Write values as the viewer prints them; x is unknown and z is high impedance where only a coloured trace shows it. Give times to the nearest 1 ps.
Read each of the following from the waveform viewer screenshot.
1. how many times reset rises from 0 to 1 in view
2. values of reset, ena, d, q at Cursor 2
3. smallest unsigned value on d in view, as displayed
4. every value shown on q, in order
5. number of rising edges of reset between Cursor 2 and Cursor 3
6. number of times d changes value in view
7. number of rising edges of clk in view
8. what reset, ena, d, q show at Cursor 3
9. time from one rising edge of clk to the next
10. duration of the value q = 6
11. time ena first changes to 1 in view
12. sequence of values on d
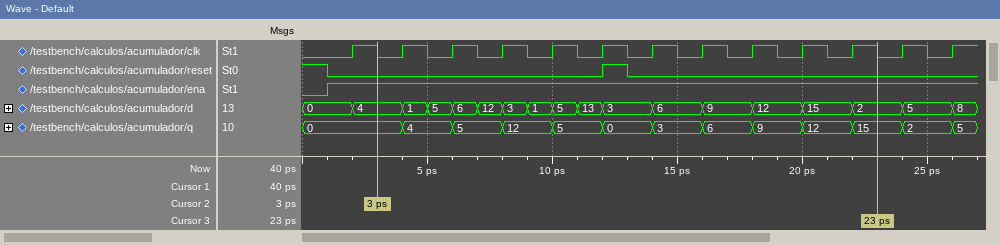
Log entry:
1
reset=0, ena=1, d=4, q=0
0
0, 4, 5, 12, 5, 0, 3, 6, 9, 12, 15, 2, 5
1
17
13
reset=0, ena=1, d=2, q=15
2 ps
2 ps
1 ps
0, 4, 1, 5, 6, 12, 3, 1, 5, 13, 3, 6, 9, 12, 15, 2, 5, 8
